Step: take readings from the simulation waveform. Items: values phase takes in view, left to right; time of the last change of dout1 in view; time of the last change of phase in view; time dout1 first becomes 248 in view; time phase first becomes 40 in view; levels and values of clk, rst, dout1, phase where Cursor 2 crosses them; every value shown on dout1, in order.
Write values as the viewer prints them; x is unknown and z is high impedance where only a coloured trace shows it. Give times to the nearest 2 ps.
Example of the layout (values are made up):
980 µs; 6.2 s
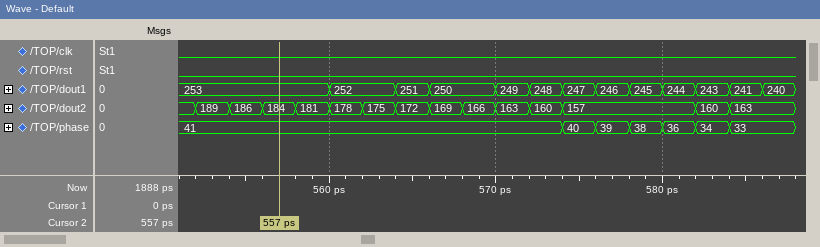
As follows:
41, 40, 39, 38, 36, 34, 33; 586 ps; 584 ps; 572 ps; 574 ps; clk=0, rst=0, dout1=253, phase=41; 253, 252, 251, 250, 249, 248, 247, 246, 245, 244, 243, 241, 240
